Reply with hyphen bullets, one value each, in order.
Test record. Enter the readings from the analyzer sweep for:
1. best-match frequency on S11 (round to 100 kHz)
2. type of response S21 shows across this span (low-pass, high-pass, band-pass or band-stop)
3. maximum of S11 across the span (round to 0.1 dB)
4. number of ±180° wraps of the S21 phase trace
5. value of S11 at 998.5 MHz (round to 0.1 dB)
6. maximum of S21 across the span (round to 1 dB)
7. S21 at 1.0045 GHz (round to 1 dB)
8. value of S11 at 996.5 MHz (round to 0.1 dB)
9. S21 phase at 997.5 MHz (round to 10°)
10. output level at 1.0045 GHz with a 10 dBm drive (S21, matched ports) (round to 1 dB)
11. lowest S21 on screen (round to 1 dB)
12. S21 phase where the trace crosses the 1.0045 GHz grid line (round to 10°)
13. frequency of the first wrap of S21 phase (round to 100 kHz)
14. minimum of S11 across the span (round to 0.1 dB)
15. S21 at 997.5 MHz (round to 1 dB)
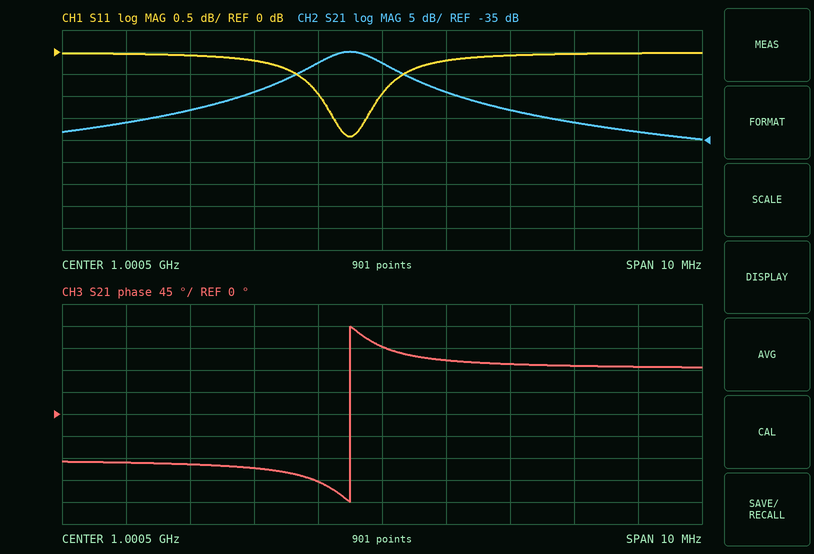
- 1.0000 GHz
- band-pass
- 0.0 dB
- 1
- -0.2 dB
- -15 dB
- -33 dB
- 0.0 dB
- -100°
- -23 dBm
- -35 dB
- 100°
- 1.0000 GHz
- -1.9 dB
- -28 dB
